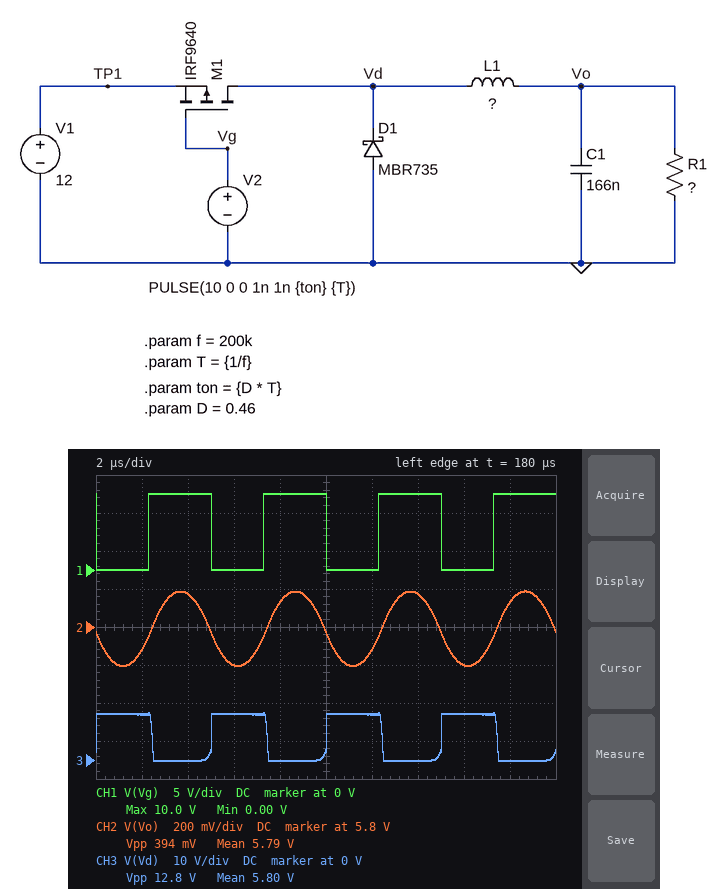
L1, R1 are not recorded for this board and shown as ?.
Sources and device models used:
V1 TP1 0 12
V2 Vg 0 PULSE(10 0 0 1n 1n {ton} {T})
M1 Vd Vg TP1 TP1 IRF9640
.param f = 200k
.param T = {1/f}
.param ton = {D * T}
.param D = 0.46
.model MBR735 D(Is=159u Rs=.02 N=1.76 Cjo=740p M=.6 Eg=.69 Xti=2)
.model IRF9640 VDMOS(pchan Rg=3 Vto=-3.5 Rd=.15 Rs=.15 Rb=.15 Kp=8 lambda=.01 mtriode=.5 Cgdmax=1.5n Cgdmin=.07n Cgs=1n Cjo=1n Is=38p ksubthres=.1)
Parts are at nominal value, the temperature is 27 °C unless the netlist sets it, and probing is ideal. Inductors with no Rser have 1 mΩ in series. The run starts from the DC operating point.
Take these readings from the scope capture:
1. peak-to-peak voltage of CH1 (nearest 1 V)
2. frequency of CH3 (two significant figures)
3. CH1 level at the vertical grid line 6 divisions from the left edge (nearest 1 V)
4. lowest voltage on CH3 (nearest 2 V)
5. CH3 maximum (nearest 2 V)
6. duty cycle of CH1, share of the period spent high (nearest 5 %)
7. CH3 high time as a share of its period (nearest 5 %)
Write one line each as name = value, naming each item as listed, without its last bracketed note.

peak-to-peak voltage of CH1 = 10 V
frequency of CH3 = 200 kHz
CH1 level at the vertical grid line 6 divisions from the left edge = 0 V
lowest voltage on CH3 = 0 V
CH3 maximum = 12 V
duty cycle of CH1, share of the period spent high = 55 %
CH3 high time as a share of its period = 50 %
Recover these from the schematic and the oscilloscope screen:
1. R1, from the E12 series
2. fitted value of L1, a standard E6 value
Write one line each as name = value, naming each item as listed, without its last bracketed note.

R1, from the E12 series = 150 Ω
fitted value of L1, a standard E6 value = 150 µH
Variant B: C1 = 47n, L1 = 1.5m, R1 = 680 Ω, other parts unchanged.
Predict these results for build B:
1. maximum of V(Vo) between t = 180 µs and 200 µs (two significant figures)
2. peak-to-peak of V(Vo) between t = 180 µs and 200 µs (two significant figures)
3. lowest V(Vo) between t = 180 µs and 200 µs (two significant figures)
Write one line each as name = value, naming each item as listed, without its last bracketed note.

maximum of V(Vo) between t = 180 µs and 200 µs = 7.2 V
peak-to-peak of V(Vo) between t = 180 µs and 200 µs = 130 mV
lowest V(Vo) between t = 180 µs and 200 µs = 7.1 V
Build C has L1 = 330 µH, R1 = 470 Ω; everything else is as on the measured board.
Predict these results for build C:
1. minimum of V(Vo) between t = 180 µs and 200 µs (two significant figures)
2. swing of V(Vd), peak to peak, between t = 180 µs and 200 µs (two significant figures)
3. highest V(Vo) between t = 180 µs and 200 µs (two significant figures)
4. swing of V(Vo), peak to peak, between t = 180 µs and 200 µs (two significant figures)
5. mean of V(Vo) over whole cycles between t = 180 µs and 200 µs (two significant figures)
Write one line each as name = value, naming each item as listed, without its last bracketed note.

minimum of V(Vo) between t = 180 µs and 200 µs = 6.2 V
swing of V(Vd), peak to peak, between t = 180 µs and 200 µs = 13 V
highest V(Vo) between t = 180 µs and 200 µs = 6.4 V
swing of V(Vo), peak to peak, between t = 180 µs and 200 µs = 170 mV
mean of V(Vo) over whole cycles between t = 180 µs and 200 µs = 6.3 V
